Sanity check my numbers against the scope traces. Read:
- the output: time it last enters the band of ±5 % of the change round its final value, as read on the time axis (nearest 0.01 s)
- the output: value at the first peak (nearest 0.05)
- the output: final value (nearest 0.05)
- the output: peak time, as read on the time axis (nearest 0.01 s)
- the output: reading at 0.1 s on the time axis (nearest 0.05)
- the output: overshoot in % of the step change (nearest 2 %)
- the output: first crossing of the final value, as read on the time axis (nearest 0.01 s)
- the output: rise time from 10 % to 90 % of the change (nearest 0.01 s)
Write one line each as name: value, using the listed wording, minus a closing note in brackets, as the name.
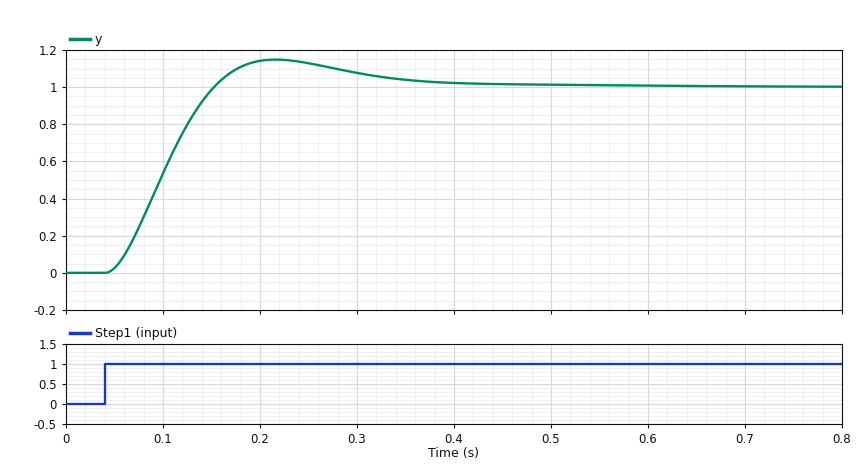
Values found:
the output: time it last enters the band of ±5 % of the change round its final value, as read on the time axis: 0.33 s
the output: value at the first peak: 1.15
the output: final value: 1.00
the output: peak time, as read on the time axis: 0.22 s
the output: reading at 0.1 s on the time axis: 0.55
the output: overshoot in % of the step change: 14 %
the output: first crossing of the final value, as read on the time axis: 0.15 s
the output: rise time from 10 % to 90 % of the change: 0.08 s
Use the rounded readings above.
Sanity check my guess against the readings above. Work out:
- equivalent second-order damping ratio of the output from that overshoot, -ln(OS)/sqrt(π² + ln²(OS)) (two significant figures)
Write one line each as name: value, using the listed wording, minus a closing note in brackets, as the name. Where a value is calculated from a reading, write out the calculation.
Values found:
equivalent second-order damping ratio of the output from that overshoot, -ln(OS)/sqrt(π² + ln²(OS)): ln(0.14) = -1.966; 1.966 / sqrt(9.870 + 3.866) = 0.53
